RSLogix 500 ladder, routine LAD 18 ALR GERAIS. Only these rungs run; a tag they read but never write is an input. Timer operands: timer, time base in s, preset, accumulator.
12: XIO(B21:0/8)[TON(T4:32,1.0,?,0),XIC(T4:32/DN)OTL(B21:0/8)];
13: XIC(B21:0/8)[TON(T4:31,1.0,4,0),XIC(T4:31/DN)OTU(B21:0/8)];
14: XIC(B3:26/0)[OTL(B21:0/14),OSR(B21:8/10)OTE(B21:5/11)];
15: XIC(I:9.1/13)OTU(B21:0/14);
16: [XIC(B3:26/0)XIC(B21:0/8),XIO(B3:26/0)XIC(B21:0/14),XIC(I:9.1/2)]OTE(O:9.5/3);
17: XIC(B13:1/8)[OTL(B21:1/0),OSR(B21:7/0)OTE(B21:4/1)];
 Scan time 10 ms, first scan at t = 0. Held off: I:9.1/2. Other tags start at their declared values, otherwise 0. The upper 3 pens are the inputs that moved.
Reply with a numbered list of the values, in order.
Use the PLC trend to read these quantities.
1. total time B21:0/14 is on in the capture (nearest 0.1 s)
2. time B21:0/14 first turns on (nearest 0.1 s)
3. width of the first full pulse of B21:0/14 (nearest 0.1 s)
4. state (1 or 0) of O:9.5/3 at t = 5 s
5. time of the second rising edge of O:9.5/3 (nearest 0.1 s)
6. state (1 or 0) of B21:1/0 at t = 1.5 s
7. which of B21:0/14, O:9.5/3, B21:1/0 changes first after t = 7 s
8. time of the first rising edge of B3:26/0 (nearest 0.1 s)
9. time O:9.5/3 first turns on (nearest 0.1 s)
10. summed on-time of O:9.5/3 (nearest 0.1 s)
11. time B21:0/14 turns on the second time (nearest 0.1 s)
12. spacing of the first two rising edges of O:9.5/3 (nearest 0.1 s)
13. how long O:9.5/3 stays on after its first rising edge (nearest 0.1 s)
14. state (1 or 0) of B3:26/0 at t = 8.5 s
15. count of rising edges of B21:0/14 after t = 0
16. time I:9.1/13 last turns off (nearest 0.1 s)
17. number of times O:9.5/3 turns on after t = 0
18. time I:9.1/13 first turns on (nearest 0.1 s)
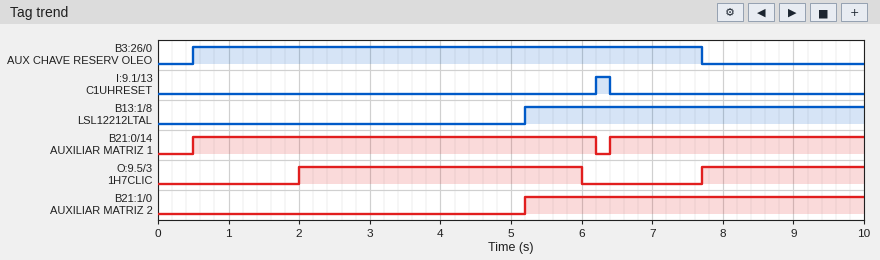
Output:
1. 9.3 s
2. 0.5 s
3. 5.7 s
4. 1
5. 7.7 s
6. 0
7. O:9.5/3
8. 0.5 s
9. 2.0 s
10. 6.3 s
11. 6.4 s
12. 5.7 s
13. 4.0 s
14. 0
15. 2
16. 6.4 s
17. 2
18. 6.2 s
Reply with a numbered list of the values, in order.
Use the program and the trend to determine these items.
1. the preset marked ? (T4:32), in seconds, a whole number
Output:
1. 2 s
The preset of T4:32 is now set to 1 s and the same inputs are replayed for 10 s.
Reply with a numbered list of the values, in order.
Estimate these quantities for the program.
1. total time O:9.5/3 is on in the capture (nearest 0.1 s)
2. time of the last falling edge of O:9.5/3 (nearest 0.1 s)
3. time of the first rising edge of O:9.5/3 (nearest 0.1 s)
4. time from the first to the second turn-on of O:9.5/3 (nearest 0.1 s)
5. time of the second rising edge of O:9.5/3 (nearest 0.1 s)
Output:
1. 8.0 s
2. 5.0 s
3. 1.0 s
4. 5.0 s
5. 6.0 s
